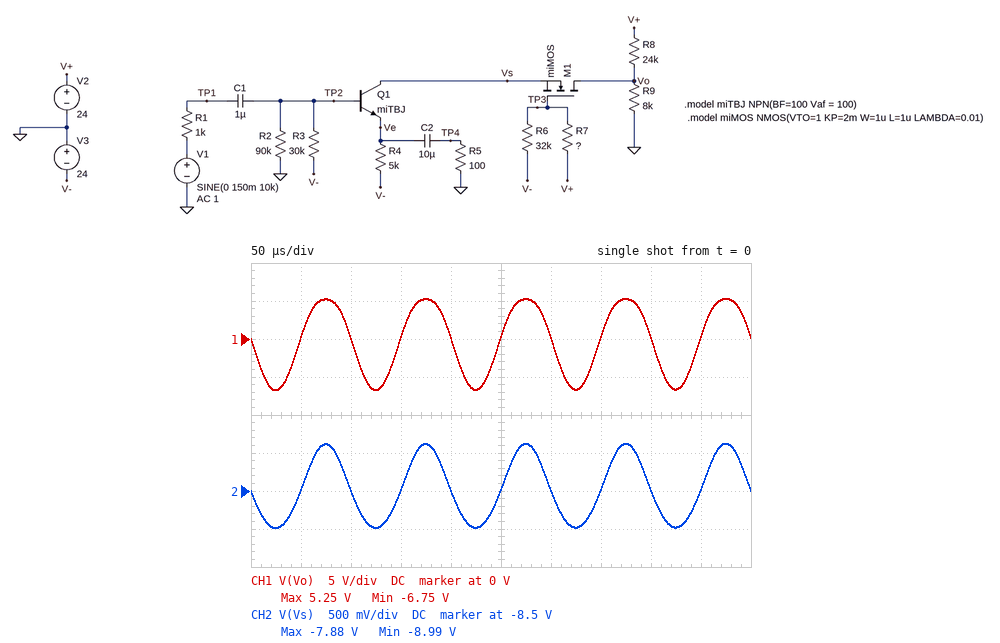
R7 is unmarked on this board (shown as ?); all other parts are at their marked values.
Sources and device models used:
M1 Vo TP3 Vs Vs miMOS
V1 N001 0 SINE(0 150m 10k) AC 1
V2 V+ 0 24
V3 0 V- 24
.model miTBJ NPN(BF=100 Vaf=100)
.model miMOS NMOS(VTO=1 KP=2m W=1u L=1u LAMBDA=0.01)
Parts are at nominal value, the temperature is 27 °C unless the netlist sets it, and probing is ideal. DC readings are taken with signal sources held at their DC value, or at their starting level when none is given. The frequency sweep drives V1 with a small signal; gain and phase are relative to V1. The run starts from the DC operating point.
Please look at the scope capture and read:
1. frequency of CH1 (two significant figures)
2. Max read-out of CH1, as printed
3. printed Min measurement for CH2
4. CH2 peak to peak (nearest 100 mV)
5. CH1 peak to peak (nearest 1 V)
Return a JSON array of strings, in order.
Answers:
["10 kHz", "5.25 V", "-8.99 V", "1.1 V", "12 V"]
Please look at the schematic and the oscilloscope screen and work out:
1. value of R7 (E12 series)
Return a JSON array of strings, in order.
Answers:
["56 kΩ"]
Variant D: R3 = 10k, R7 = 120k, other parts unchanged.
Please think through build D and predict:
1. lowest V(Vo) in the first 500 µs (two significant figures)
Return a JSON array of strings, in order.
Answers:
["-1.4 V"]
